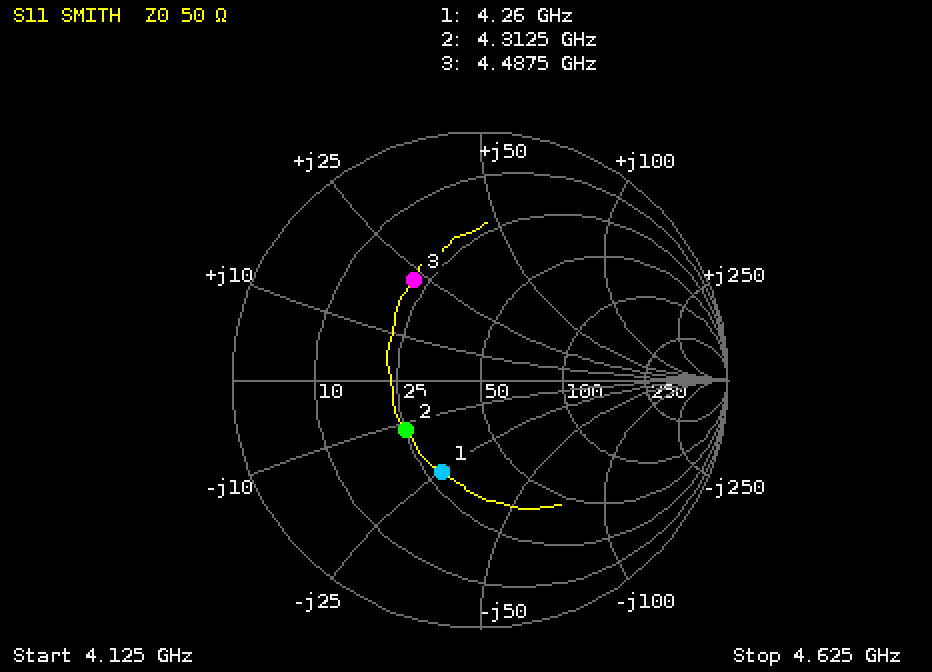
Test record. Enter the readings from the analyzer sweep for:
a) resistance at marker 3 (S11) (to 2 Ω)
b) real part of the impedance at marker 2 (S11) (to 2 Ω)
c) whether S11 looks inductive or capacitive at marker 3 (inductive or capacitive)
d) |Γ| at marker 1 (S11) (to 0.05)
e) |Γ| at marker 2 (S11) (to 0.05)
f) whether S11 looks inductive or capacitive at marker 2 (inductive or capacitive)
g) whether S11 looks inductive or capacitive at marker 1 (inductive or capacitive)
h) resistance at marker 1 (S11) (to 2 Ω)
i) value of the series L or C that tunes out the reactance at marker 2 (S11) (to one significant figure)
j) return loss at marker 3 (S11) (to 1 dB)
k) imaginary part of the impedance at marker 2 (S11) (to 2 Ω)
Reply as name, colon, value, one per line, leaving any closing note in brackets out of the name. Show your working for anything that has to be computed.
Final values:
resistance at marker 3 (S11): 22 Ω
real part of the impedance at marker 2 (S11): 26 Ω
whether S11 looks inductive or capacitive at marker 3: inductive
|Γ| at marker 1 (S11): 0.40
|Γ| at marker 2 (S11): 0.35
whether S11 looks inductive or capacitive at marker 2: capacitive
whether S11 looks inductive or capacitive at marker 1: capacitive
resistance at marker 1 (S11): 28 Ω
value of the series L or C that tunes out the reactance at marker 2 (S11): L = 12 Ω/(2π × 4.3125 GHz) ≈ 443 pH, so 400 pH to one significant figure
return loss at marker 3 (S11): 6 dB
imaginary part of the impedance at marker 2 (S11): -12 Ω
